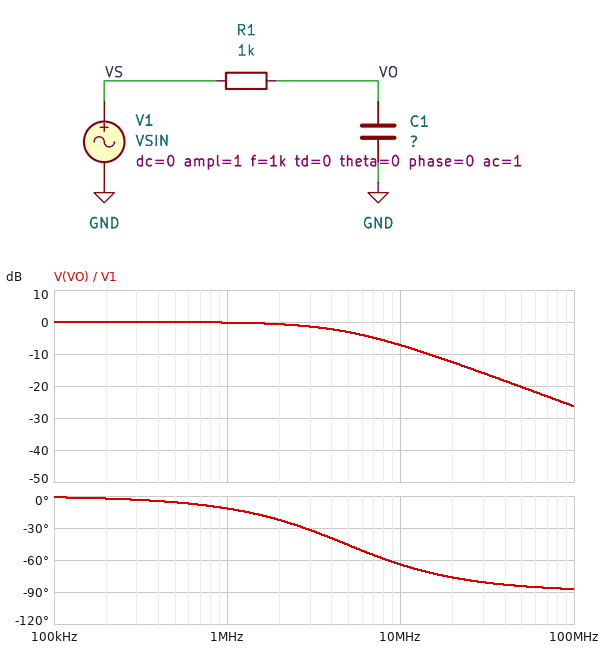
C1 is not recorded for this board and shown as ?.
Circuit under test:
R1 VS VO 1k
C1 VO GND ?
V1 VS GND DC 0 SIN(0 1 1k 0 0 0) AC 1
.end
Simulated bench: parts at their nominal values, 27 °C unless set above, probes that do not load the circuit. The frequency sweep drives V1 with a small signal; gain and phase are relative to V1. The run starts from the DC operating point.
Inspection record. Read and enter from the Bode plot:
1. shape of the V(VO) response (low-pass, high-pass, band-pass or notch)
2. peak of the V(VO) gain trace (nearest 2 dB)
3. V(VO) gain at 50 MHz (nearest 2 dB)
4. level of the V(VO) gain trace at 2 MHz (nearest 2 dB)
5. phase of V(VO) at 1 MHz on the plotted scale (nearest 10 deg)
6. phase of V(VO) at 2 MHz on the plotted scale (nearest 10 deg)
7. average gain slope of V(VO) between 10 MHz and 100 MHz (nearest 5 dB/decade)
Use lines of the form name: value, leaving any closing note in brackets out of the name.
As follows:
shape of the V(VO) response: low-pass
peak of the V(VO) gain trace: 0 dB
V(VO) gain at 50 MHz: -20 dB
level of the V(VO) gain trace at 2 MHz: 0 dB
phase of V(VO) at 1 MHz on the plotted scale: -10 deg
phase of V(VO) at 2 MHz on the plotted scale: -20 deg
average gain slope of V(VO) between 10 MHz and 100 MHz: -20 dB/decade
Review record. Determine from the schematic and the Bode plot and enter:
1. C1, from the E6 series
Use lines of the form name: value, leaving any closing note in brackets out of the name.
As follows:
C1, from the E6 series: 33 pF
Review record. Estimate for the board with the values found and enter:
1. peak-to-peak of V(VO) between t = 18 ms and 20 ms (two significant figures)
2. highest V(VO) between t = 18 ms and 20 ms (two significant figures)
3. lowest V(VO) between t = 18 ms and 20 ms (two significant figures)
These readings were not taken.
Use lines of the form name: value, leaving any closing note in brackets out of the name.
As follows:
peak-to-peak of V(VO) between t = 18 ms and 20 ms: 2.0 V
highest V(VO) between t = 18 ms and 20 ms: 1.0 V
lowest V(VO) between t = 18 ms and 20 ms: -1.0 V
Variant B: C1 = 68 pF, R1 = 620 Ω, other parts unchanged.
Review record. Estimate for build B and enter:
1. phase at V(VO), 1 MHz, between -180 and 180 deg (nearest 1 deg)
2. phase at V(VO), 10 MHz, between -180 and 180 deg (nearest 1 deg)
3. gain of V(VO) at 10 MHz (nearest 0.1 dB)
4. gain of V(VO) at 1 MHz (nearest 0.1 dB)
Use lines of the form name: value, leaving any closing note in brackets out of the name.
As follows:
phase at V(VO), 1 MHz, between -180 and 180 deg: -15 deg
phase at V(VO), 10 MHz, between -180 and 180 deg: -69 deg
gain of V(VO) at 10 MHz: -9.0 dB
gain of V(VO) at 1 MHz: -0.3 dB
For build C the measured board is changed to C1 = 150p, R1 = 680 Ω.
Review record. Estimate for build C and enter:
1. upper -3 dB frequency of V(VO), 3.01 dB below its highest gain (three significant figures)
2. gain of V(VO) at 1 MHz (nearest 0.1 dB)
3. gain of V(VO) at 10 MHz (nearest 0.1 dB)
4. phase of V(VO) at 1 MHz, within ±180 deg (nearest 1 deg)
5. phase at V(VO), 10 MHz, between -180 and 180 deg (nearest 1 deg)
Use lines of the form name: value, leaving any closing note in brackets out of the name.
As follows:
upper -3 dB frequency of V(VO), 3.01 dB below its highest gain: 1.56 MHz
gain of V(VO) at 1 MHz: -1.5 dB
gain of V(VO) at 10 MHz: -16.2 dB
phase of V(VO) at 1 MHz, within ±180 deg: -33 deg
phase at V(VO), 10 MHz, between -180 and 180 deg: -81 deg
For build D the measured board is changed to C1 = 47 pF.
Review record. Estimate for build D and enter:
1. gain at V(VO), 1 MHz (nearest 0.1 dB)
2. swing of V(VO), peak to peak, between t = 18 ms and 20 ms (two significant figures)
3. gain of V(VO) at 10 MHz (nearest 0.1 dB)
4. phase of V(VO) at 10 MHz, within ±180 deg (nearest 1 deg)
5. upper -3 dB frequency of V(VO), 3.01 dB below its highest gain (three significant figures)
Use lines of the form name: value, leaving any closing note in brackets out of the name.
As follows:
gain at V(VO), 1 MHz: -0.4 dB
swing of V(VO), peak to peak, between t = 18 ms and 20 ms: 2.0 V
gain of V(VO) at 10 MHz: -9.9 dB
phase of V(VO) at 10 MHz, within ±180 deg: -71 deg
upper -3 dB frequency of V(VO), 3.01 dB below its highest gain: 3.39 MHz
